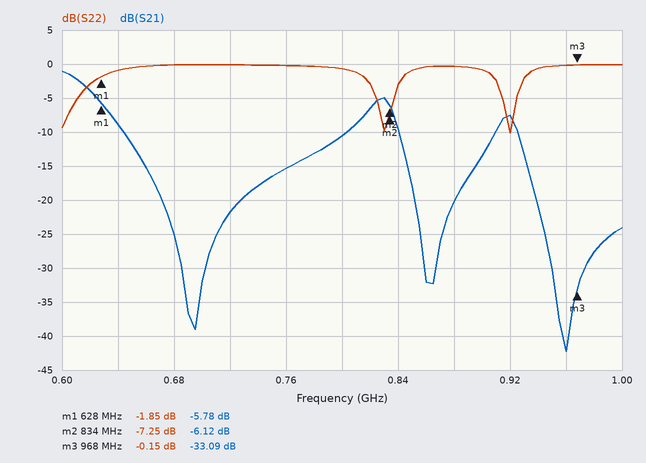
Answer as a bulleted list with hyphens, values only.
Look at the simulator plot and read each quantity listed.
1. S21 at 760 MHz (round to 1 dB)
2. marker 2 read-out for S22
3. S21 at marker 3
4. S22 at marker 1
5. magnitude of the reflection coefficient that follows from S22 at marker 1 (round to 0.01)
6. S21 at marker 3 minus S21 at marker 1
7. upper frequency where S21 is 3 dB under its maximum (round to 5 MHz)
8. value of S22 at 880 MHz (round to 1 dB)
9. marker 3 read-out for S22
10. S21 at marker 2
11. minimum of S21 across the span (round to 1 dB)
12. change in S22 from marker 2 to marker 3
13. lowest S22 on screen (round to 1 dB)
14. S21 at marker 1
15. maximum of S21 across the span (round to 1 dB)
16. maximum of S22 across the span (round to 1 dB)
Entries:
- -15 dB
- -7.25 dB
- -33.09 dB
- -1.85 dB
- 0.81
- -27.31 dB
- 620 MHz
- 0 dB
- -0.15 dB
- -6.12 dB
- -42 dB
- 7.10 dB
- -10 dB
- -5.78 dB
- -1 dB
- 0 dB
